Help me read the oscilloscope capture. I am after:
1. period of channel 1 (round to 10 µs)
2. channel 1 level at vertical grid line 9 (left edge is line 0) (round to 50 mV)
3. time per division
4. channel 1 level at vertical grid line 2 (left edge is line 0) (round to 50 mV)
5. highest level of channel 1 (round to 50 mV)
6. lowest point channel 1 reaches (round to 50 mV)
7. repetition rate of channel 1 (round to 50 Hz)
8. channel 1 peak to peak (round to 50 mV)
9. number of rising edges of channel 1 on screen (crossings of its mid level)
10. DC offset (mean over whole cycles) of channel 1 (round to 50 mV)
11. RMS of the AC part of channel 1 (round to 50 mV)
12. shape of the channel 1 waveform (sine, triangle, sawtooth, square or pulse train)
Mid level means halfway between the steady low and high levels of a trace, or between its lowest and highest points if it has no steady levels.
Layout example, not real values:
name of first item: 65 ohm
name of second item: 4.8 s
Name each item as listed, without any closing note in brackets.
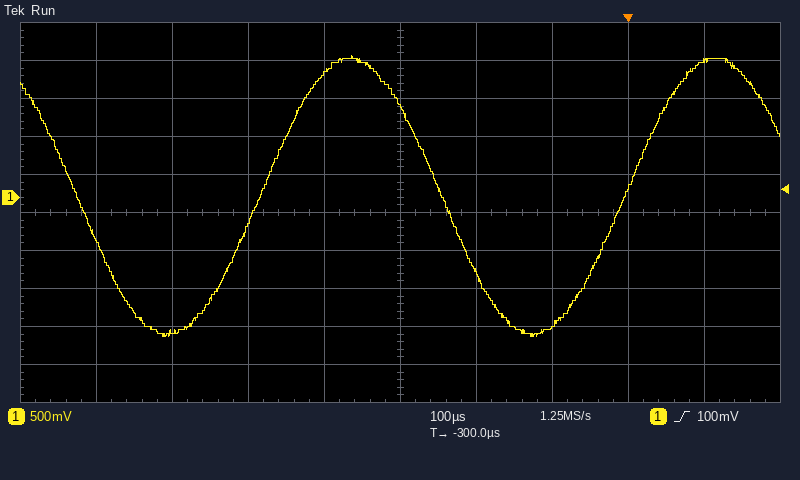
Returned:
period of channel 1: 480 µs
channel 1 level at vertical grid line 9 (left edge is line 0): 1.80 V
time per division: 100 µs
channel 1 level at vertical grid line 2 (left edge is line 0): -1.80 V
highest level of channel 1: 1.85 V
lowest point channel 1 reaches: -1.85 V
repetition rate of channel 1: 2.10 kHz
channel 1 peak to peak: 3.70 V
number of rising edges of channel 1 on screen: 2
DC offset (mean over whole cycles) of channel 1: 0 mV
RMS of the AC part of channel 1: 1.30 V
shape of the channel 1 waveform: sine
